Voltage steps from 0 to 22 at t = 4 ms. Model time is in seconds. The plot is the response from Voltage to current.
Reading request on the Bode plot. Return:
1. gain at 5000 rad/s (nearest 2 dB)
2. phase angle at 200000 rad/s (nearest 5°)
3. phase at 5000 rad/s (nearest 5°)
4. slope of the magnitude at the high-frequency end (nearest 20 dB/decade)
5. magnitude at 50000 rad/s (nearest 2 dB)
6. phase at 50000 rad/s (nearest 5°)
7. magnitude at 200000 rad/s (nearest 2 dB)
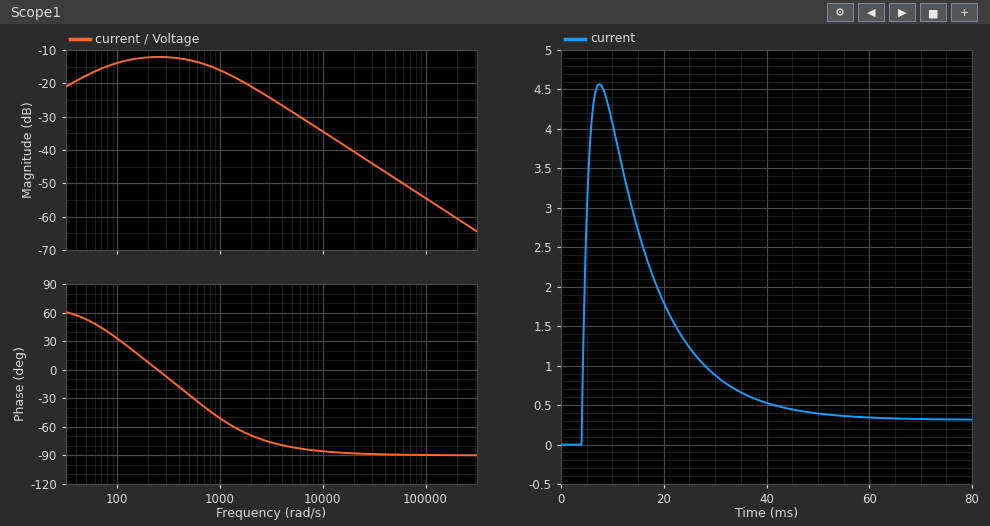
-28 dB
-90°
-80°
-20 dB/decade
-48 dB
-90°
-60 dB
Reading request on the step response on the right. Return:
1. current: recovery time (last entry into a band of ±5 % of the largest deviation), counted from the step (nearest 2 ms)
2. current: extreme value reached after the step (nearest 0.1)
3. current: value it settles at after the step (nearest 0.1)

36 ms
4.6
0.3
